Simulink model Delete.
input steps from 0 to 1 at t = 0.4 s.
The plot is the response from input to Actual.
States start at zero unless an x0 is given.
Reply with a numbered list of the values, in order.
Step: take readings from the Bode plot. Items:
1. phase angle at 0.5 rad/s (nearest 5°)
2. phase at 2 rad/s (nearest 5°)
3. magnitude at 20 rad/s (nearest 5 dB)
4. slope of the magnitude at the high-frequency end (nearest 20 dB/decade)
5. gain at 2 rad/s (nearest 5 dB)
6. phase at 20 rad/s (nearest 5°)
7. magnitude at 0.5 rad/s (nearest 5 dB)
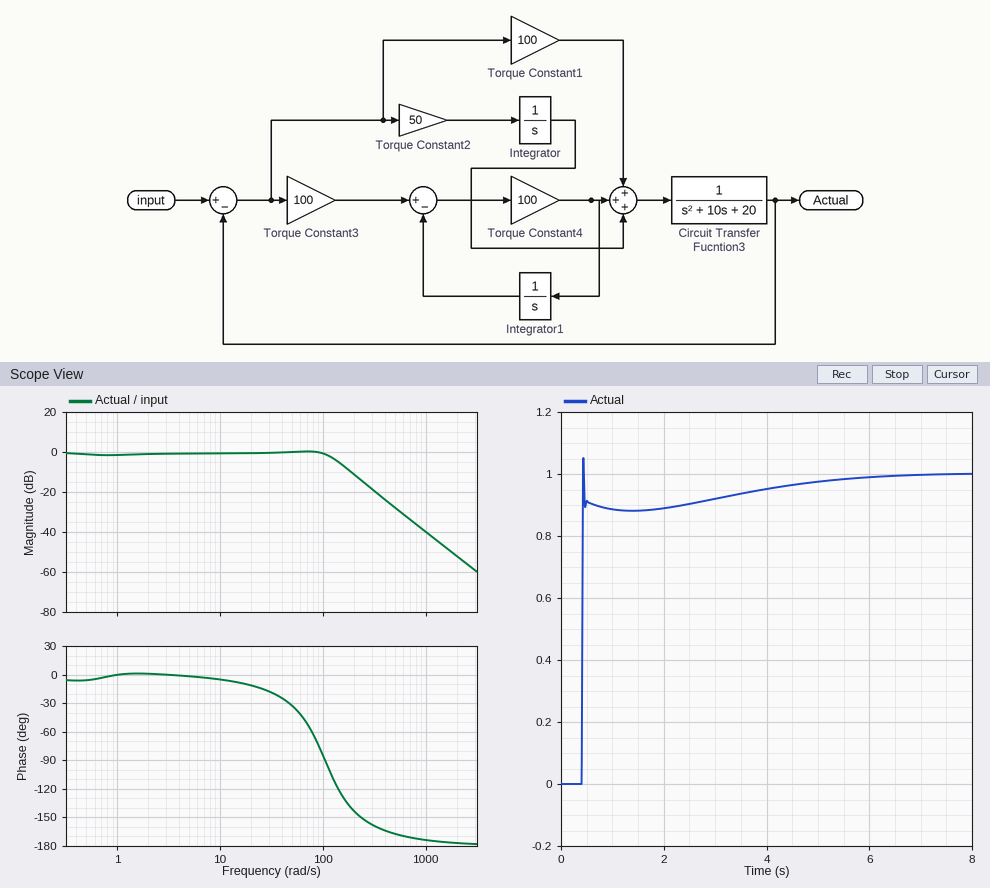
1. -5°
2. 0°
3. 0 dB
4. -40 dB/decade
5. 0 dB
6. -10°
7. 0 dB
